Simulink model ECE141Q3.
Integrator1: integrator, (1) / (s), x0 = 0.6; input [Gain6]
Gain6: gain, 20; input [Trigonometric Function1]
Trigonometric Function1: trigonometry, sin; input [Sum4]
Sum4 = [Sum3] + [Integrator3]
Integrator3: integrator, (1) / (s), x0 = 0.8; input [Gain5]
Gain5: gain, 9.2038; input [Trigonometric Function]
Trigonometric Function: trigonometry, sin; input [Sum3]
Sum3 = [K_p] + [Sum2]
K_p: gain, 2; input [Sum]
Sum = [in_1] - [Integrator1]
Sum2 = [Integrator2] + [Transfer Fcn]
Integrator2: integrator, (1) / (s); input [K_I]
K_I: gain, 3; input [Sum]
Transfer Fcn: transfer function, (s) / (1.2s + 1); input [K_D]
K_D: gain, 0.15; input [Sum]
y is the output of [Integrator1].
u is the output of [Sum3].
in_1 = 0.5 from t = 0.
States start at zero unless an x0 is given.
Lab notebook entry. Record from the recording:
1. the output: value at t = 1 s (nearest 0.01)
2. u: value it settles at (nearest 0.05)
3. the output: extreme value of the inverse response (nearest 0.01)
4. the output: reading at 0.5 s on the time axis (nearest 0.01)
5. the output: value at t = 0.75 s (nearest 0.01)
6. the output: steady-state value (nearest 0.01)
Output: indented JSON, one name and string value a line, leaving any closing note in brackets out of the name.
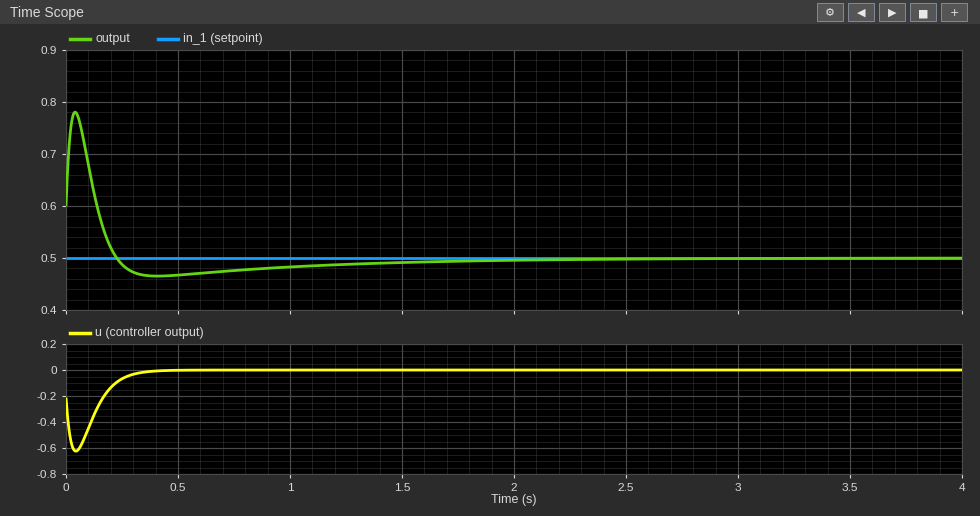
{
  "the output: value at t = 1 s": "0.48",
  "u: value it settles at": "0.00",
  "the output: extreme value of the inverse response": "0.78",
  "the output: reading at 0.5 s on the time axis": "0.47",
  "the output: value at t = 0.75 s": "0.48",
  "the output: steady-state value": "0.50"
}
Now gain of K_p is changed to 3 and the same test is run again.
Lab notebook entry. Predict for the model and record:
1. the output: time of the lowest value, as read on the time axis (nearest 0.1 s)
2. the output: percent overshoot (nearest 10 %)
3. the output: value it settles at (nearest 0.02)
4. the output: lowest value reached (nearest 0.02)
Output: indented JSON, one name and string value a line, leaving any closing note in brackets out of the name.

{
  "the output: time of the lowest value, as read on the time axis": "0.5 s",
  "the output: percent overshoot": "20 %",
  "the output: value it settles at": "0.50",
  "the output: lowest value reached": "0.48"
}
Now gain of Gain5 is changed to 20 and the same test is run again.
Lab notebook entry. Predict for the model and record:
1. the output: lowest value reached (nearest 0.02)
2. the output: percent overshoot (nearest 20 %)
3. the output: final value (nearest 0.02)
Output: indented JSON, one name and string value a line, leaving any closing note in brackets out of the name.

{
  "the output: lowest value reached": "0.46",
  "the output: percent overshoot": "40 %",
  "the output: final value": "0.50"
}
